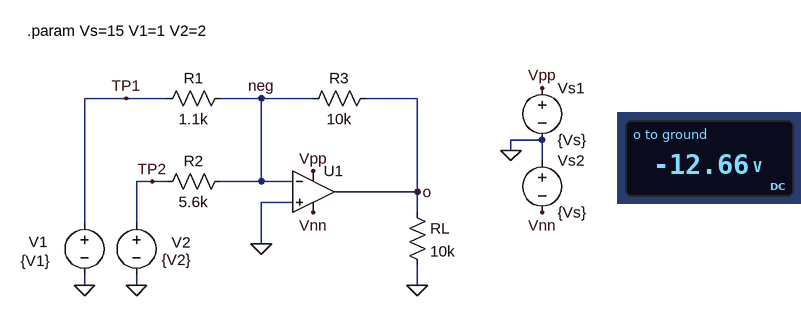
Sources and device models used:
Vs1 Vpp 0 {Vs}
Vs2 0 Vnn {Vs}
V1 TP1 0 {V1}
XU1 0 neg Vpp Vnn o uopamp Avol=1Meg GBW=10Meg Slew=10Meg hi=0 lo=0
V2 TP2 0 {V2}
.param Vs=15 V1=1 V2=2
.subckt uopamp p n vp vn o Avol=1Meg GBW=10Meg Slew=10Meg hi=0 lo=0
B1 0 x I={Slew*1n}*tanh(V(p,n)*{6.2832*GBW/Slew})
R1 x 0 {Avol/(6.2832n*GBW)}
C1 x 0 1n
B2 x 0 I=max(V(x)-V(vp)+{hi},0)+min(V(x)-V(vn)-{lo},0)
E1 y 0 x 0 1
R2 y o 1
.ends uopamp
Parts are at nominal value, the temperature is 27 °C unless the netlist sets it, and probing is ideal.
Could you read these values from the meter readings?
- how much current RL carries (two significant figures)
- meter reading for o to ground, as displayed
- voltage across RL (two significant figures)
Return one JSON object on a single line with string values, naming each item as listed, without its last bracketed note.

{"how much current RL carries": "1.3 mA", "meter reading for o to ground, as displayed": "-12.66 V", "voltage across RL": "13 V"}
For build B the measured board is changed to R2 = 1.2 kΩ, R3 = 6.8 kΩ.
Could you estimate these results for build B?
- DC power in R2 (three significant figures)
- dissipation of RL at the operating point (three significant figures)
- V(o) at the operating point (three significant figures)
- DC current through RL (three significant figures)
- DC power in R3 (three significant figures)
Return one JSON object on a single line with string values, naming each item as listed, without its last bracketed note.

{"DC power in R2": "2.71 mW", "dissipation of RL at the operating point": "22.5 mW", "V(o) at the operating point": "-15.0 V", "DC current through RL": "1.50 mA", "DC power in R3": "34.0 mW"}
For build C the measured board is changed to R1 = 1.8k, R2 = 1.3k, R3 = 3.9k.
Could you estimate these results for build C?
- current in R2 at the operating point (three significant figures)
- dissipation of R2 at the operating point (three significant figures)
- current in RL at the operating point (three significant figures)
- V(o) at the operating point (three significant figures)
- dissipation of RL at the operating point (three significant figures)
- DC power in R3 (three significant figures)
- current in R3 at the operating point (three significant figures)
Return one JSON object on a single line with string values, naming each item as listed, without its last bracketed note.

{"current in R2 at the operating point": "1.54 mA", "dissipation of R2 at the operating point": "3.08 mW", "current in RL at the operating point": "817 µA", "V(o) at the operating point": "-8.17 V", "dissipation of RL at the operating point": "6.67 mW", "DC power in R3": "17.1 mW", "current in R3 at the operating point": "2.09 mA"}
